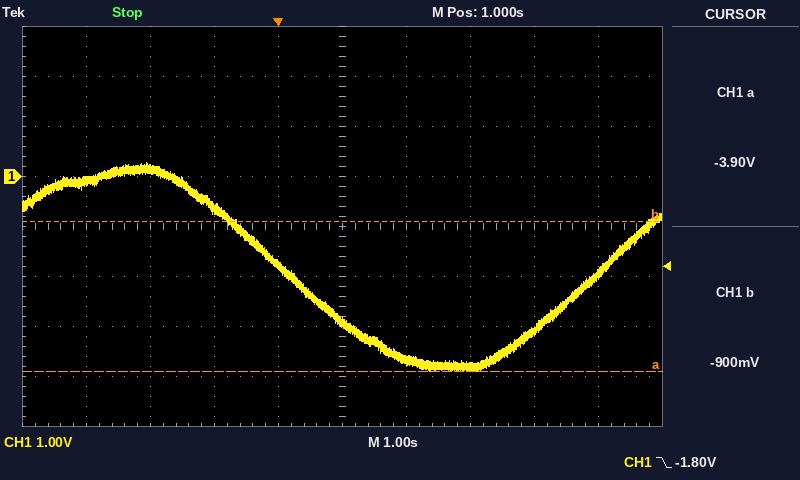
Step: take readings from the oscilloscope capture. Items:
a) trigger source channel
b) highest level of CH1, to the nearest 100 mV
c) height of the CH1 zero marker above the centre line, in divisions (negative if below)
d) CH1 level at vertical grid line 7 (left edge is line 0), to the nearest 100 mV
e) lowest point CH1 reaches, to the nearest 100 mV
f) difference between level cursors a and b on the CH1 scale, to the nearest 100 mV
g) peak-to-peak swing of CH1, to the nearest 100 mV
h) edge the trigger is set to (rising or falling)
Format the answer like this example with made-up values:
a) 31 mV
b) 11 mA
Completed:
a) CH1
b) 300 mV
c) +1.0 div
d) -3.8 V
e) -3.9 V
f) 3.0 V
g) 4.2 V
h) falling
